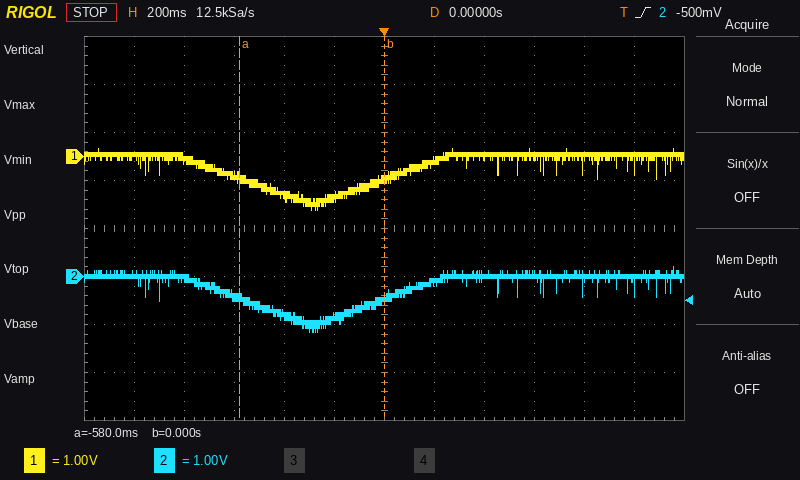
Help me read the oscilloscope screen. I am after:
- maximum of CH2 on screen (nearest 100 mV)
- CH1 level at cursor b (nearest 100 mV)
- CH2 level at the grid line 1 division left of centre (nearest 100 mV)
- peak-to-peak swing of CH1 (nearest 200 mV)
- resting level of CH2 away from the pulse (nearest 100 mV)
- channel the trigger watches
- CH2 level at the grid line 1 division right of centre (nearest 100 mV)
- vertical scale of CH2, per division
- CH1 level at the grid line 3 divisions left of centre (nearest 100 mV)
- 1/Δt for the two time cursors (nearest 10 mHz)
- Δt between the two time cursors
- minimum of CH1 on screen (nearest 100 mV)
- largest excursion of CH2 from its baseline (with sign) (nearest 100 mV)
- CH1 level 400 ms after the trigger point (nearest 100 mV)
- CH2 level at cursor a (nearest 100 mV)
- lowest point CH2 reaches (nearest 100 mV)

200 mV
-500 mV
-800 mV
1.2 V
0.0 V
CH2
-100 mV
1 V
-400 mV
1.72 Hz
580 ms
-1.1 V
-1.2 V
0.0 V
-400 mV
-1.2 V
